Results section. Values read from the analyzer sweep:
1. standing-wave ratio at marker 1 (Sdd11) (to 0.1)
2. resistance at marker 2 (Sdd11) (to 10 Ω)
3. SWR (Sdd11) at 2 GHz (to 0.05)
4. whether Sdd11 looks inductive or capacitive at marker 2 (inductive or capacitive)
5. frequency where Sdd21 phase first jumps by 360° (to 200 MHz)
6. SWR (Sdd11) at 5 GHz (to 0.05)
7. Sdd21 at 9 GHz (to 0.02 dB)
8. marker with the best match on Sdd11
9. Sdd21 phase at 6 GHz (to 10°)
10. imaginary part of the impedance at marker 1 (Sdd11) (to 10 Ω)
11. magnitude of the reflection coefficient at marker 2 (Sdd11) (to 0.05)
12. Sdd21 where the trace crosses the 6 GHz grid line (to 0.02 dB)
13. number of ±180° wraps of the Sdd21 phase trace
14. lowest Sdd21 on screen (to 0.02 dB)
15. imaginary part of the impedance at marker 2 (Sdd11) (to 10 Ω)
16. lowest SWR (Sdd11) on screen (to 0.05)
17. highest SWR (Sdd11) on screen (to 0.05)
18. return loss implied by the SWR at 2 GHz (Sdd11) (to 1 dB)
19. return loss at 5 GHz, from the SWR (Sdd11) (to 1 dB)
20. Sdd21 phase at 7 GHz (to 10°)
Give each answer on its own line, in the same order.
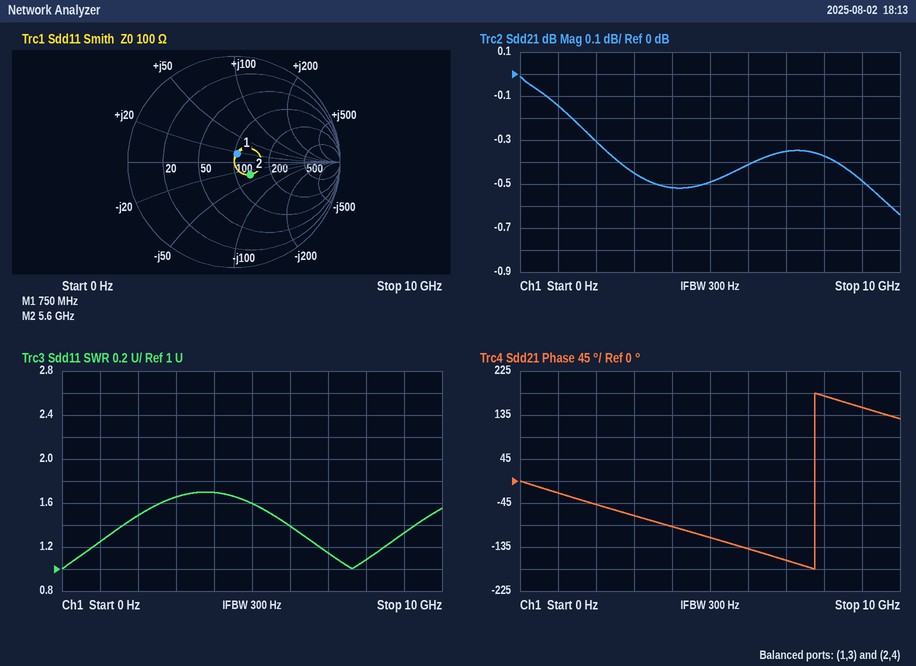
1.2
130 Ω
1.50
capacitive
7.8 GHz
1.60
-0.48 dB
marker 1
-140°
+20 Ω
0.20
-0.42 dB
1
-0.64 dB
-30 Ω
1.00
1.70
14 dB
13 dB
-160°
